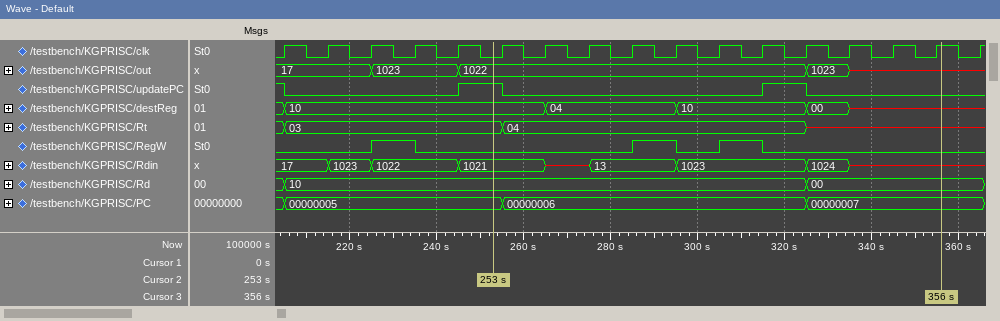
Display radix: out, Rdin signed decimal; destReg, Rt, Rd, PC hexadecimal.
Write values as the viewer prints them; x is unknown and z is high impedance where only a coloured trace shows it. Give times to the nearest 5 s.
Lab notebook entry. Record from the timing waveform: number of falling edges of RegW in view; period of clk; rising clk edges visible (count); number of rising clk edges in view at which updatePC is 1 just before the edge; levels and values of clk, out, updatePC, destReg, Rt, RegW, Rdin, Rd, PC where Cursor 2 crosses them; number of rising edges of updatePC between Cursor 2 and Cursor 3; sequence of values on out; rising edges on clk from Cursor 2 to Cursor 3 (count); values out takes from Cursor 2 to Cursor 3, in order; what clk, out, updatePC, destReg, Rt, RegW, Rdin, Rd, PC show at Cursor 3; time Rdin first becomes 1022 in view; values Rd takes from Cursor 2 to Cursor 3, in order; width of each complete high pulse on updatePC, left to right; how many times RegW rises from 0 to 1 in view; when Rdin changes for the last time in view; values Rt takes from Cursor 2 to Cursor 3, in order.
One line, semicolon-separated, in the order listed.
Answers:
3; 10 s; 17; 3; clk=0, out=1022, updatePC=1, destReg=10, Rt=03, RegW=0, Rdin=1021, Rd=10, PC=00000005; 1; 17, 1023, 1022, 1023, x; 11; 1022, 1023, x; clk=1, out=x, updatePC=0, destReg=x, Rt=x, RegW=0, Rdin=x, Rd=00, PC=00000007; 225 s; 10, 00; 10 s, 10 s; 3; 335 s; 03, 04, x
